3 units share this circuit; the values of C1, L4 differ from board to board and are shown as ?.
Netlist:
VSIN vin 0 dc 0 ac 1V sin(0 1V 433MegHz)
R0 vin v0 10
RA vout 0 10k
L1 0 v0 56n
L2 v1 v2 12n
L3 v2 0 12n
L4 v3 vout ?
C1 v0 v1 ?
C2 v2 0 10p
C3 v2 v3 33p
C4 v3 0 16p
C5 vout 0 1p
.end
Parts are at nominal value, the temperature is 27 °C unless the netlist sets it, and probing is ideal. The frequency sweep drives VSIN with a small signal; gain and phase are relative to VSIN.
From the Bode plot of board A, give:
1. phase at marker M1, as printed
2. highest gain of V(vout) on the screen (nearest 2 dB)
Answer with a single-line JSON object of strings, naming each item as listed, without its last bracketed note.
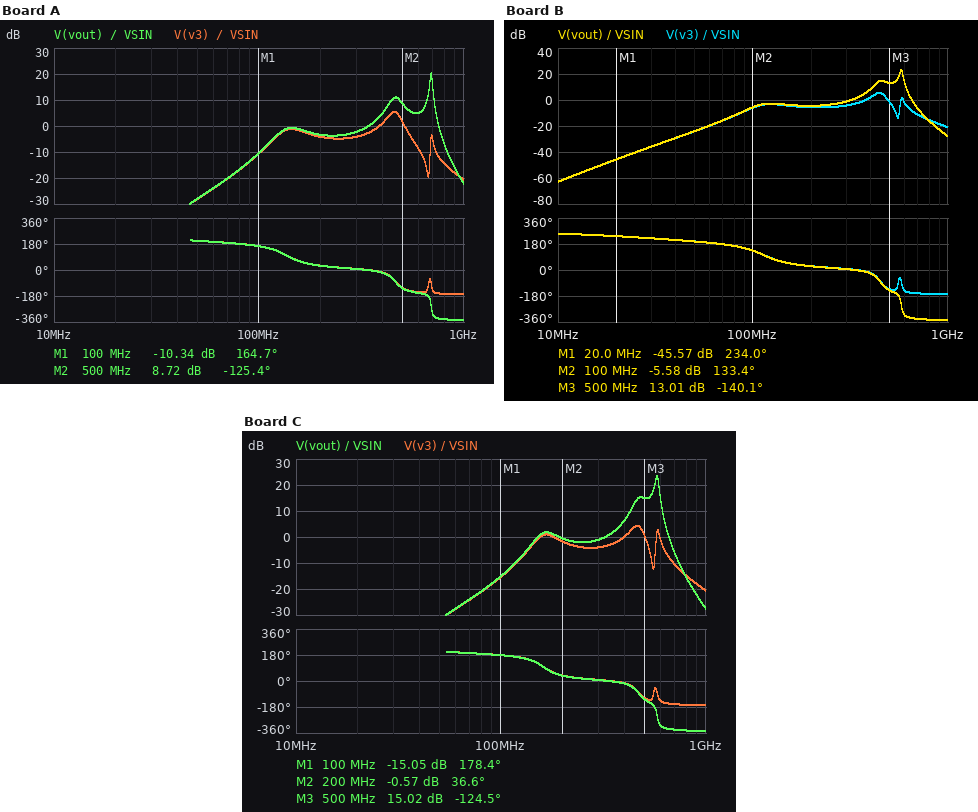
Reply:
{"phase at marker M1, as printed": "164.7 deg", "highest gain of V(vout) on the screen": "20 dB"}
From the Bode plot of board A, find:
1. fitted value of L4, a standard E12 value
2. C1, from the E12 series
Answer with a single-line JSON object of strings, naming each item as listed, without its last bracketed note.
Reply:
{"fitted value of L4, a standard E12 value": "56 nH", "C1, from the E12 series": "47 pF"}
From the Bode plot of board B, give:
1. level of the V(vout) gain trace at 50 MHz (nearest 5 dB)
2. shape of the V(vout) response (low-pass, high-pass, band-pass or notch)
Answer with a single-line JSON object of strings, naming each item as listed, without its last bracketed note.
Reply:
{"level of the V(vout) gain trace at 50 MHz": "-25 dB", "shape of the V(vout) response": "band-pass"}
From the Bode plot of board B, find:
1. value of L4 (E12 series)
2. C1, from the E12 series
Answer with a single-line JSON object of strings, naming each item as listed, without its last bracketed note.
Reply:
{"value of L4": "82 nH", "C1, from the E12 series": "68 pF"}
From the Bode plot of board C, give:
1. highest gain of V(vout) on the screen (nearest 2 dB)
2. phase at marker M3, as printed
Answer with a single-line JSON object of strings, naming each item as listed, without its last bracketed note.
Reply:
{"highest gain of V(vout) on the screen": "24 dB", "phase at marker M3, as printed": "-124.5 deg"}
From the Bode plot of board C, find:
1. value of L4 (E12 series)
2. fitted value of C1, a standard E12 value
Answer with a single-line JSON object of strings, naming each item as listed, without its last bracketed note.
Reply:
{"value of L4": "82 nH", "fitted value of C1, a standard E12 value": "33 pF"}
